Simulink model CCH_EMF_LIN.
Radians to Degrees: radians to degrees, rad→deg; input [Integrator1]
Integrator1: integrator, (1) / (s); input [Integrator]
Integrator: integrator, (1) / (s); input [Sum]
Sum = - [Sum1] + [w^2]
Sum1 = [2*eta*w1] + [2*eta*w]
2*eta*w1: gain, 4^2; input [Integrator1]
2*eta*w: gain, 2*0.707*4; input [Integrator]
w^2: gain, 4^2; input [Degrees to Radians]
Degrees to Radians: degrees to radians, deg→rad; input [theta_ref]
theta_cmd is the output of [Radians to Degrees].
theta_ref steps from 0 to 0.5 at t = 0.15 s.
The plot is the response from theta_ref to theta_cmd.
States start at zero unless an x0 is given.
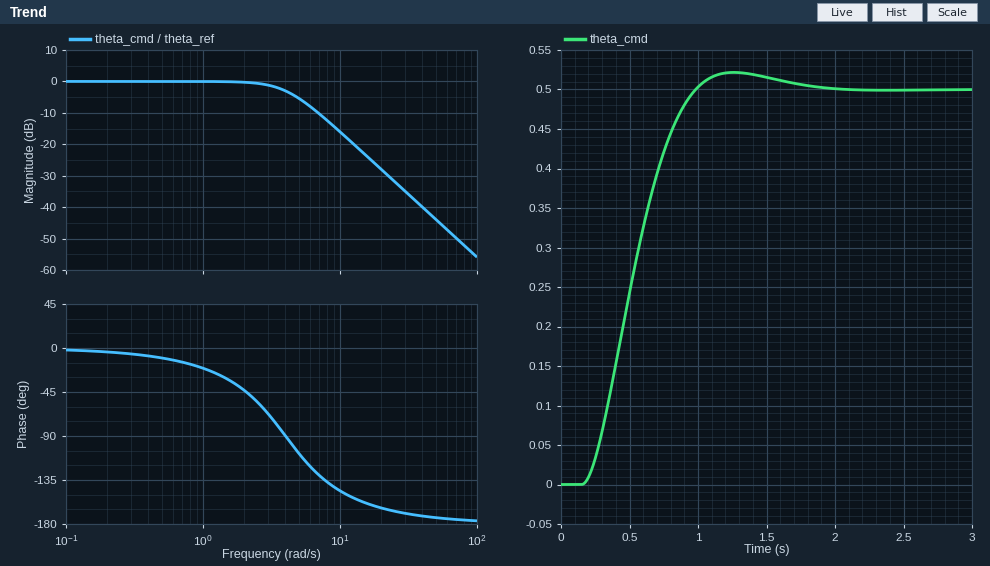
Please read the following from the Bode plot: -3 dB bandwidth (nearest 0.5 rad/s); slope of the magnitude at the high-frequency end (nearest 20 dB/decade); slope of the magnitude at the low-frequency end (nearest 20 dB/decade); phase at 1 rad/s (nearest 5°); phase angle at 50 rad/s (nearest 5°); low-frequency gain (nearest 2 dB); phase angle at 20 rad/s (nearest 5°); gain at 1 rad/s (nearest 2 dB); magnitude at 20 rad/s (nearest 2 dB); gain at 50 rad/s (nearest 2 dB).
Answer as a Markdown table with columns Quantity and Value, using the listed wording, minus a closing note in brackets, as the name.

| Quantity | Value |
|---|---|
| -3 dB bandwidth | 4.0 rad/s |
| slope of the magnitude at the high-frequency end | -40 dB/decade |
| slope of the magnitude at the low-frequency end | 0 dB/decade |
| phase at 1 rad/s | -20° |
| phase angle at 50 rad/s | -175° |
| low-frequency gain | 0 dB |
| phase angle at 20 rad/s | -165° |
| gain at 1 rad/s | 0 dB |
| magnitude at 20 rad/s | -28 dB |
| gain at 50 rad/s | -44 dB |
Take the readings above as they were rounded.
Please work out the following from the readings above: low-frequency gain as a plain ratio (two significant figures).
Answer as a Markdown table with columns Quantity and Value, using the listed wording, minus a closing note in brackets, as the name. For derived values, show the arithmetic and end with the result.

| Quantity | Value |
|---|---|
| low-frequency gain as a plain ratio | 10^(0 / 20) = 1.0 |
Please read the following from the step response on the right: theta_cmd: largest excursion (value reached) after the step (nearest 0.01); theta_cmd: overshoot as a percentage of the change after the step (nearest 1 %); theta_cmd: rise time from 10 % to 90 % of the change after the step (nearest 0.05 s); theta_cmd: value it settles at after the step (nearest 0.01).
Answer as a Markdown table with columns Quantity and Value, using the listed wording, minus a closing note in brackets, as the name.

| Quantity | Value |
|---|---|
| theta_cmd: largest excursion (value reached) after the step | 0.52 |
| theta_cmd: overshoot as a percentage of the change after the step | 4 % |
| theta_cmd: rise time from 10 % to 90 % of the change after the step | 0.55 s |
| theta_cmd: value it settles at after the step | 0.50 |
